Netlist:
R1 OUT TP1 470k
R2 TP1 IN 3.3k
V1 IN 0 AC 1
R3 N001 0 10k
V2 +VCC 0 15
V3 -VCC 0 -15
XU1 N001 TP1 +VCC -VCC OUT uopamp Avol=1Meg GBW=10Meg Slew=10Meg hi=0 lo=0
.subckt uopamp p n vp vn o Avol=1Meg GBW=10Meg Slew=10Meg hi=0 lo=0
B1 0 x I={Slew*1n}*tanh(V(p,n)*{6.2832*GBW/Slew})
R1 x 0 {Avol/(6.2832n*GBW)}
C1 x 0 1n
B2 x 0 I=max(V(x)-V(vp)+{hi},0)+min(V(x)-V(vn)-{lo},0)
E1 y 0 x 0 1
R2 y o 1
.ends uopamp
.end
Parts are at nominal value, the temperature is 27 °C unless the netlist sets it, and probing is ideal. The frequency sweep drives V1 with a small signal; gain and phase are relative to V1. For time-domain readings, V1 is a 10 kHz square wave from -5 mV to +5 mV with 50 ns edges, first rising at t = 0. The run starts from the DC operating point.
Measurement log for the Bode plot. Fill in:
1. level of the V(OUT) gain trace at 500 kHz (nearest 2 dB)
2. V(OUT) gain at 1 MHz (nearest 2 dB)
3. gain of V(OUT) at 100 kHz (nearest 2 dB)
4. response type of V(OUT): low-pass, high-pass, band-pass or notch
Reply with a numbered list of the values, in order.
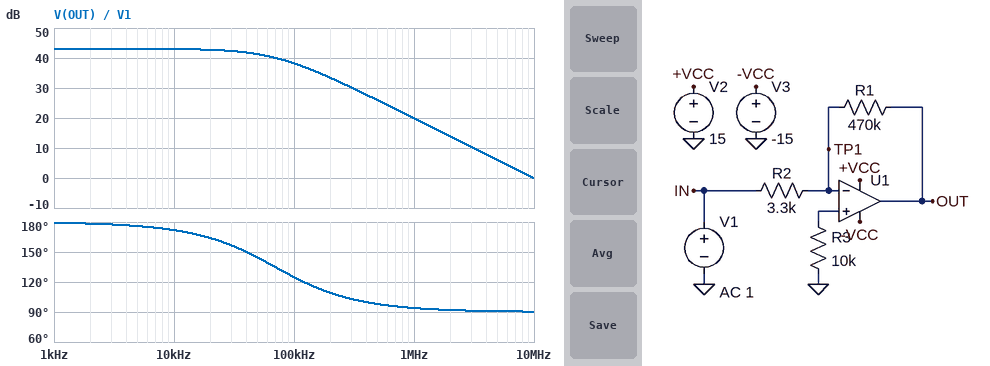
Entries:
1. 26 dB
2. 20 dB
3. 38 dB
4. low-pass
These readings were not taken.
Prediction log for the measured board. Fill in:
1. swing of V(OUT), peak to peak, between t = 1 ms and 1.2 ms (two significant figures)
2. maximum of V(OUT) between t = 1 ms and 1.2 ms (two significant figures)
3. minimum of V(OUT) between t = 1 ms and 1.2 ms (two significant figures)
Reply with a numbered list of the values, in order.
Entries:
1. 1.4 V
2. 710 mV
3. -710 mV
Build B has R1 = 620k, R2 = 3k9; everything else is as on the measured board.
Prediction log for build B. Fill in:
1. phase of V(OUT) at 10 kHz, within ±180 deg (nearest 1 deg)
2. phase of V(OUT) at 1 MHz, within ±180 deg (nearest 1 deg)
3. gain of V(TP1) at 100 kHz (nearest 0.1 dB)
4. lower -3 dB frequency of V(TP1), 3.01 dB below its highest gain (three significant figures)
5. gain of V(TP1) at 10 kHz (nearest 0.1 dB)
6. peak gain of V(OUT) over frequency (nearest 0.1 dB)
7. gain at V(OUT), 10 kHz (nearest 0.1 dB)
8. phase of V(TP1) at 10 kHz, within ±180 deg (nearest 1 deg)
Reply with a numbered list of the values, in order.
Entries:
1. 171 deg
2. 94 deg
3. -1.5 dB
4. 62.5 kHz
5. -16.1 dB
6. 44.0 dB
7. 43.9 dB
8. 81 deg
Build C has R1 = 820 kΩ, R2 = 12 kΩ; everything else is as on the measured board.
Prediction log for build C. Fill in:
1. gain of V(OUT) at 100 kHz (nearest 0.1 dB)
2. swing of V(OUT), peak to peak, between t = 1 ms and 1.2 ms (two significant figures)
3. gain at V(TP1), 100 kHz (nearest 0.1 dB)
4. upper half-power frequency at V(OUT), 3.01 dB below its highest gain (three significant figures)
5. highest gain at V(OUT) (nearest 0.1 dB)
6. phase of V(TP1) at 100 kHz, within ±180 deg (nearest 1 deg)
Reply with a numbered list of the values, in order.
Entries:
1. 35.0 dB
2. 680 mV
3. -5.0 dB
4. 144 kHz
5. 36.7 dB
6. 55 deg
